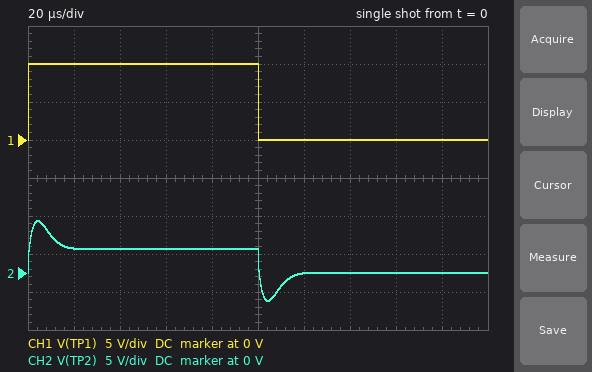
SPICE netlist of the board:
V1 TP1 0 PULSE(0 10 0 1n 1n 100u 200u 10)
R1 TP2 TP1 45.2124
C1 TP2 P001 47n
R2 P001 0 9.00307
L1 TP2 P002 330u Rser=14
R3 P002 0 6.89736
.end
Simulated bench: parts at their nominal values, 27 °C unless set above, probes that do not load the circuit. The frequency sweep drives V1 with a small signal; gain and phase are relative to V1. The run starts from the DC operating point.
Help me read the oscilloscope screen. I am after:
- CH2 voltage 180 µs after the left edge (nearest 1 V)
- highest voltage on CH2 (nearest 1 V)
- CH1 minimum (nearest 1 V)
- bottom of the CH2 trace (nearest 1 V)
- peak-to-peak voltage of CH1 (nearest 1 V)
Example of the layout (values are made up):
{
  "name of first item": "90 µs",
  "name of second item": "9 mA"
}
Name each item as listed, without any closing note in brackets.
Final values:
{
  "CH2 voltage 180 µs after the left edge": "0 V",
  "highest voltage on CH2": "7 V",
  "CH1 minimum": "0 V",
  "bottom of the CH2 trace": "-4 V",
  "peak-to-peak voltage of CH1": "10 V"
}
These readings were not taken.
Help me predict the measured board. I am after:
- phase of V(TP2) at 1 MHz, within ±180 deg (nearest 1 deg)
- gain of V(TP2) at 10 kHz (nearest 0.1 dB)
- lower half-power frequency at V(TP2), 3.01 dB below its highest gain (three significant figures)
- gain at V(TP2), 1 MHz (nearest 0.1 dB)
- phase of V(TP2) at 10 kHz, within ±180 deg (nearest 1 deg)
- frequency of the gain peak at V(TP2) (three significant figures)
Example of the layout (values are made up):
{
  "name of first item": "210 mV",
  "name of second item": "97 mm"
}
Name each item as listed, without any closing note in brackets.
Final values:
{
  "phase of V(TP2) at 1 MHz, within ±180 deg": "-17 deg",
  "gain of V(TP2) at 10 kHz": "-7.2 dB",
  "lower half-power frequency at V(TP2), 3.01 dB below its highest gain": "18.1 kHz",
  "gain at V(TP2), 1 MHz": "-15.0 dB",
  "phase of V(TP2) at 10 kHz, within ±180 deg": "24 deg",
  "frequency of the gain peak at V(TP2)": "43.4 kHz"
}
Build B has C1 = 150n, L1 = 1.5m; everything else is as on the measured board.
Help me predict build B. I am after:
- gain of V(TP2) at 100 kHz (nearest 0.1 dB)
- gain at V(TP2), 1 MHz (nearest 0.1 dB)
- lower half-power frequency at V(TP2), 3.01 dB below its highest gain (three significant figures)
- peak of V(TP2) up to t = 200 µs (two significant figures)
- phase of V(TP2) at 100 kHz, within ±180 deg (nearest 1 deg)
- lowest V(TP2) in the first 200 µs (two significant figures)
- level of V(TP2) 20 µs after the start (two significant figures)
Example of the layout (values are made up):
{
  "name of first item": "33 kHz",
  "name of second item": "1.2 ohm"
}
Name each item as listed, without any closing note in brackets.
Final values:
{
  "gain of V(TP2) at 100 kHz": "-11.9 dB",
  "gain at V(TP2), 1 MHz": "-15.5 dB",
  "lower half-power frequency at V(TP2), 3.01 dB below its highest gain": "4.41 kHz",
  "peak of V(TP2) up to t = 200 µs": "7.3 V",
  "phase of V(TP2) at 100 kHz, within ±180 deg": "-38 deg",
  "lowest V(TP2) in the first 200 µs": "-4.1 V",
  "level of V(TP2) 20 µs after the start": "7.1 V"
}
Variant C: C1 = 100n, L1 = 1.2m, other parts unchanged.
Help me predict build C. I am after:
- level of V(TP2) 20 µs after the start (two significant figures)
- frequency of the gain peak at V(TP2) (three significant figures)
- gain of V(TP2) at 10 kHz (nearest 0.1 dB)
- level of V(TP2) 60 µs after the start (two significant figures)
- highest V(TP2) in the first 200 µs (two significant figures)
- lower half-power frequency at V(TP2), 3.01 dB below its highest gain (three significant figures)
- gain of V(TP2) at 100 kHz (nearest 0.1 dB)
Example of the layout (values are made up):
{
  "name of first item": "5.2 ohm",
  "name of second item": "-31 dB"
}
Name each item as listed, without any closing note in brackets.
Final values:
{
  "level of V(TP2) 20 µs after the start": "6.5 V",
  "frequency of the gain peak at V(TP2)": "15.7 kHz",
  "gain of V(TP2) at 10 kHz": "-1.6 dB",
  "level of V(TP2) 60 µs after the start": "3.4 V",
  "highest V(TP2) in the first 200 µs": "7.5 V",
  "lower half-power frequency at V(TP2), 3.01 dB below its highest gain": "5.78 kHz",
  "gain of V(TP2) at 100 kHz": "-9.7 dB"
}
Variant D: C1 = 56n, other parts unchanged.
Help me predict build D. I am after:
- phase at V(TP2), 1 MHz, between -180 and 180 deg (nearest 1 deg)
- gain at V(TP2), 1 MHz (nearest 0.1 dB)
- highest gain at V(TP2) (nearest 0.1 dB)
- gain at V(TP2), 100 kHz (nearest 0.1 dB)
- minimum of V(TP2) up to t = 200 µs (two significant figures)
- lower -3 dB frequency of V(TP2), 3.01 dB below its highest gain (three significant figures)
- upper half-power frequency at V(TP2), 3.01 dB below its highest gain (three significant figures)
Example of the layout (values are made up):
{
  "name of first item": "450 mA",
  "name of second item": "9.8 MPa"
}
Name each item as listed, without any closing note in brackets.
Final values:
{
  "phase at V(TP2), 1 MHz, between -180 and 180 deg": "-14 deg",
  "gain at V(TP2), 1 MHz": "-15.2 dB",
  "highest gain at V(TP2)": "-1.7 dB",
  "gain at V(TP2), 100 kHz": "-5.7 dB",
  "minimum of V(TP2) up to t = 200 µs": "-3.5 V",
  "lower -3 dB frequency of V(TP2), 3.01 dB below its highest gain": "17.0 kHz",
  "upper half-power frequency at V(TP2), 3.01 dB below its highest gain": "86.1 kHz"
}
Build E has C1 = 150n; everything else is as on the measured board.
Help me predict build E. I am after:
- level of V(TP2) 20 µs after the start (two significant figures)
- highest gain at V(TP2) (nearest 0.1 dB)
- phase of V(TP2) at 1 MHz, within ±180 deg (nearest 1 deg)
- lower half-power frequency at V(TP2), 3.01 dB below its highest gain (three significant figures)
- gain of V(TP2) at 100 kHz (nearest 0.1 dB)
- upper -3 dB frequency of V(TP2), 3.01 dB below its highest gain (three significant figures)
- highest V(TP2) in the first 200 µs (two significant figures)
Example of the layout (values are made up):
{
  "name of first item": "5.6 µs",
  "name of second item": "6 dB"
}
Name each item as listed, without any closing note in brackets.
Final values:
{
  "level of V(TP2) 20 µs after the start": "3.9 V",
  "highest gain at V(TP2)": "-3.7 dB",
  "phase of V(TP2) at 1 MHz, within ±180 deg": "-5 deg",
  "lower half-power frequency at V(TP2), 3.01 dB below its highest gain": "10.5 kHz",
  "gain of V(TP2) at 100 kHz": "-11.7 dB",
  "upper -3 dB frequency of V(TP2), 3.01 dB below its highest gain": "46.4 kHz",
  "highest V(TP2) in the first 200 µs": "5.3 V"
}
